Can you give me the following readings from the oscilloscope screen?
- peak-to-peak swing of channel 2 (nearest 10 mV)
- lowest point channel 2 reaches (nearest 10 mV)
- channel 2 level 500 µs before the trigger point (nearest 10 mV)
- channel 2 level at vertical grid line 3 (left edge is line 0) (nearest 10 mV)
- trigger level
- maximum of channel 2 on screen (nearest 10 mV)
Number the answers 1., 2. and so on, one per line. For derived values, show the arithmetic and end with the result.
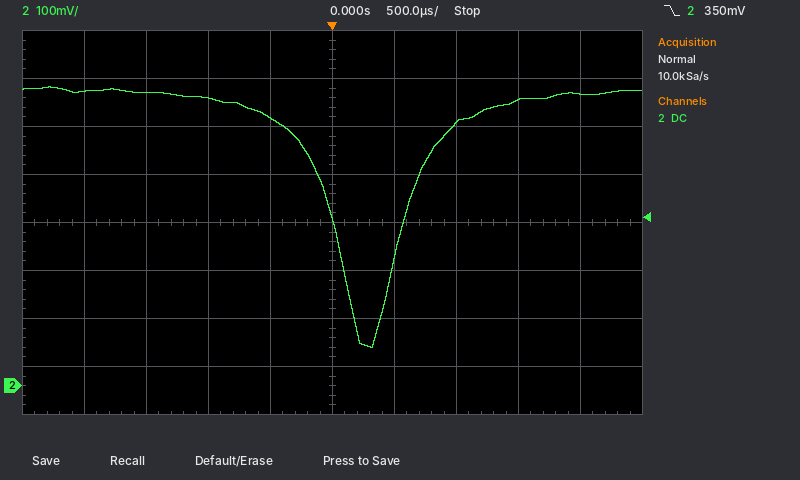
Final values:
1. 620 mV − (80 mV) = 540 mV
2. 80 mV
3. 560 mV
4. 600 mV
5. 350 mV
6. 620 mV
